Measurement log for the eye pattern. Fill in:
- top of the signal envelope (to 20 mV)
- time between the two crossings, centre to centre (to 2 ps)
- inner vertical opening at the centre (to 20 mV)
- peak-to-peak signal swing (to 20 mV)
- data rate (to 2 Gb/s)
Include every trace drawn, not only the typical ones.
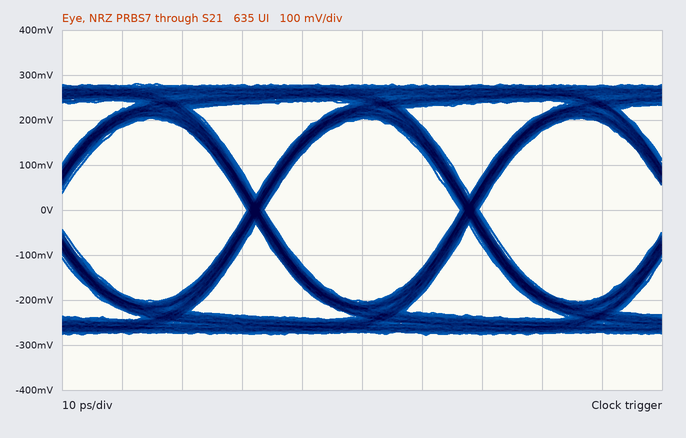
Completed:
280 mV
36 ps
400 mV
560 mV
28 Gb/s
